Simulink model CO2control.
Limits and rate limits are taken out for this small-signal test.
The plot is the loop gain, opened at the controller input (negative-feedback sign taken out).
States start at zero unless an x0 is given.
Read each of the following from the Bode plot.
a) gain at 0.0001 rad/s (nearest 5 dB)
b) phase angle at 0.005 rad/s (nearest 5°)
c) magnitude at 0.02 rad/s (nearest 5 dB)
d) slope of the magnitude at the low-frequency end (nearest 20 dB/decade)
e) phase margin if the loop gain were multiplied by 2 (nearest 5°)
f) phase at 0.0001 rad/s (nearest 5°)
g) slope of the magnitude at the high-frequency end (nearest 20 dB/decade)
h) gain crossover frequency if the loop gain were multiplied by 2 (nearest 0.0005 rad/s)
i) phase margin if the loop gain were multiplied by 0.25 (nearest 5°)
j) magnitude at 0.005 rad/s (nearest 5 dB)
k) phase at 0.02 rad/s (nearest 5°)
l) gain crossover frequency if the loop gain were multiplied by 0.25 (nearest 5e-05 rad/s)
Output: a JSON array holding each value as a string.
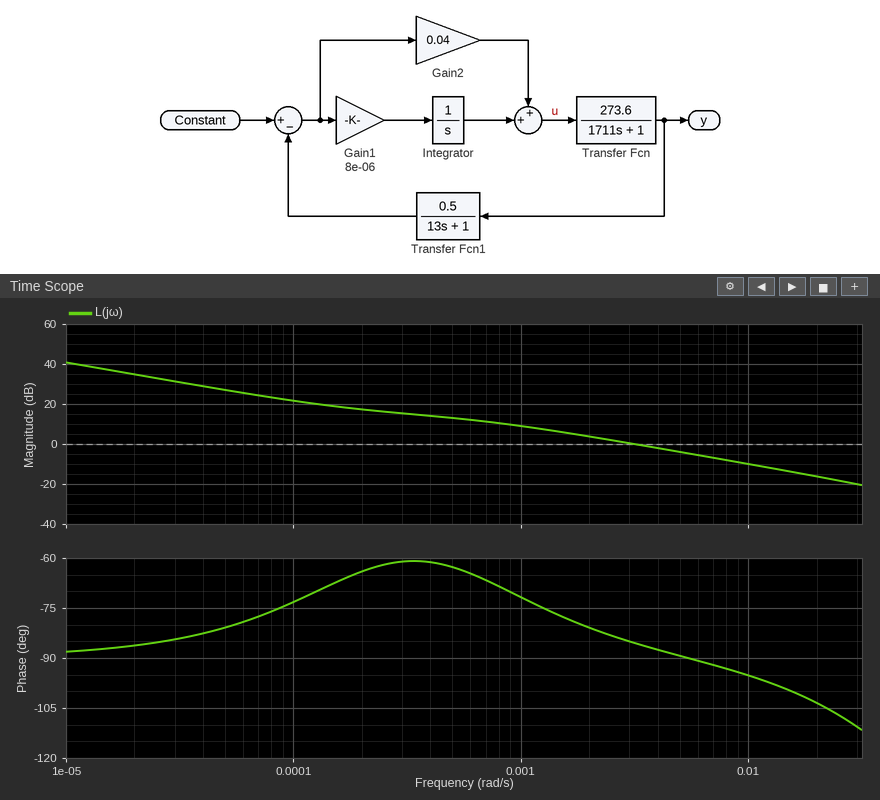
["20 dB", "-90°", "-15 dB", "-20 dB/decade", "90°", "-75°", "-20 dB/decade", "0.0065 rad/s", "115°", "-5 dB", "-105°", "0.00060 rad/s"]
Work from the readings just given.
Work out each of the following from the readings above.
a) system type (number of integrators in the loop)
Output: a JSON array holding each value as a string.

["1"]
